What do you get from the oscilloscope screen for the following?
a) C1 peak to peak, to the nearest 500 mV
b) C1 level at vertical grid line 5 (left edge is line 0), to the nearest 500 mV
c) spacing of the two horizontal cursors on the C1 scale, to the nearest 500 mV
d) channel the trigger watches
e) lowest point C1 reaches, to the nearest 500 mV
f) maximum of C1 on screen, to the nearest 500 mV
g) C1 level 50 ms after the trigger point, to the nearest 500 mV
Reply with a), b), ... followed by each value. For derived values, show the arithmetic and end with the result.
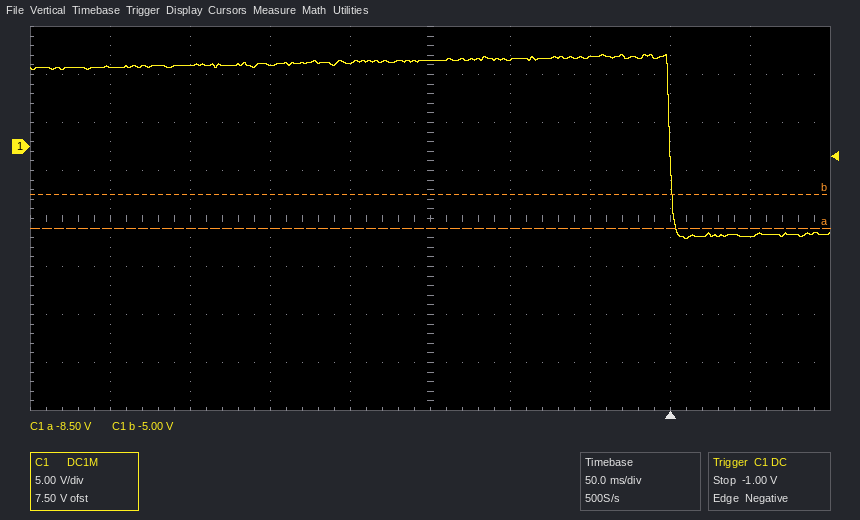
a) 9.5 V − (-9.5 V) = 19.0 V
b) 9.0 V
c) 3.5 V
d) C1
e) -9.5 V
f) 9.5 V
g) -9.5 V
